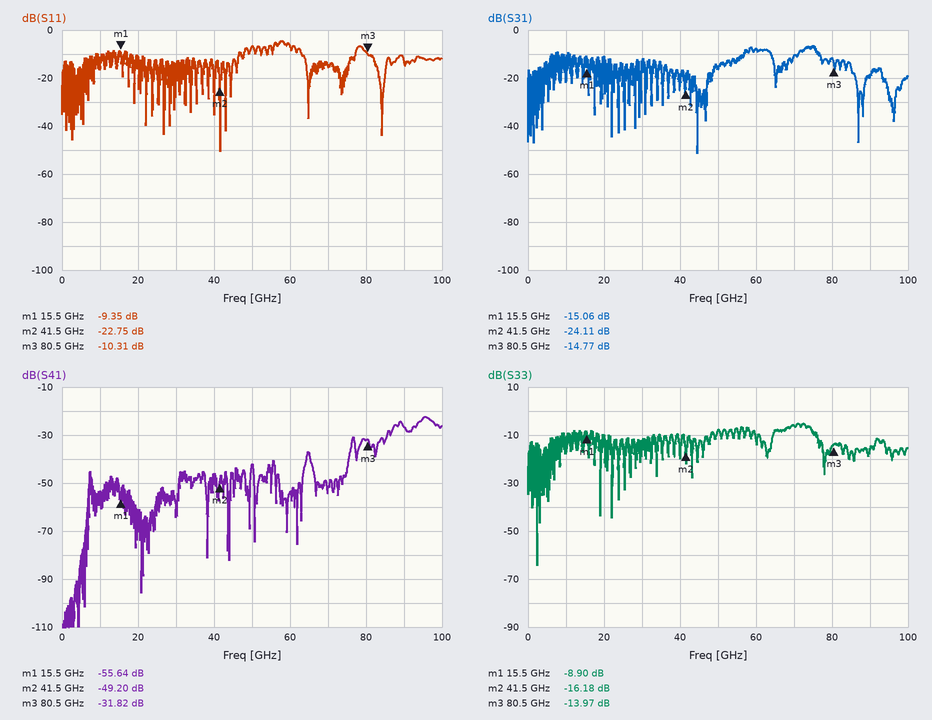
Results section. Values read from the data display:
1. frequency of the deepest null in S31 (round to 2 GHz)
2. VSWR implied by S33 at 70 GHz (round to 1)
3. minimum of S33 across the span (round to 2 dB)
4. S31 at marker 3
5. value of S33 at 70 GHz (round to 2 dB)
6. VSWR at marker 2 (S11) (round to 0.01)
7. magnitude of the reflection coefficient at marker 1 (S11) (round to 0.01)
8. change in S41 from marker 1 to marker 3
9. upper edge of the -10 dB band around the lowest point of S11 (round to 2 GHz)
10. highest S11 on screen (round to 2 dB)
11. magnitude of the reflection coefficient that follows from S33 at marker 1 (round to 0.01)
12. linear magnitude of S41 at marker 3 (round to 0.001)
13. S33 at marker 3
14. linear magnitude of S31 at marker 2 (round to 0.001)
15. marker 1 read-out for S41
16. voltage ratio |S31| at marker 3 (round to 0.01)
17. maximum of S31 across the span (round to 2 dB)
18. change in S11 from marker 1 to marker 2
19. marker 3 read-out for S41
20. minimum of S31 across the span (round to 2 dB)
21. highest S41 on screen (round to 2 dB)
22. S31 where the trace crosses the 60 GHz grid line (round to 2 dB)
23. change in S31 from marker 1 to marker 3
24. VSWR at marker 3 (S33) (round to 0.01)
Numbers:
44 GHz
3
-64 dB
-14.77 dB
-6 dB
1.16
0.34
23.82 dB
46 GHz
-4 dB
0.36
0.026
-13.97 dB
0.062
-55.64 dB
0.18
-6 dB
-13.40 dB
-31.82 dB
-52 dB
-22 dB
-8 dB
0.29 dB
1.50
